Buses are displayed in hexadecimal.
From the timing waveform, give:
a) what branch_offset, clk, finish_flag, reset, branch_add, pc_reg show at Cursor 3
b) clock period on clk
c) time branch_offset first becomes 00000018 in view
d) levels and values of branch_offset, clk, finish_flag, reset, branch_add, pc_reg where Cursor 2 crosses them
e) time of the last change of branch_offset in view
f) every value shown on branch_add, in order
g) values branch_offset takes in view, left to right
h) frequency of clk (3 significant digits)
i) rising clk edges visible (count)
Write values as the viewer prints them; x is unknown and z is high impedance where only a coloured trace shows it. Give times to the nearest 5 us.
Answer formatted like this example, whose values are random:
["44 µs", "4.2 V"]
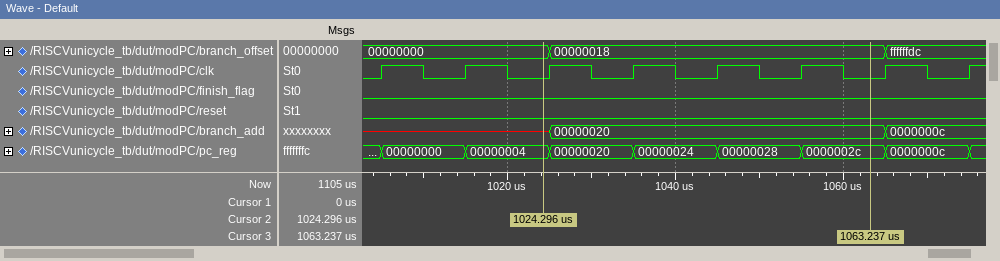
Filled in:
["branch_offset=00000018, clk=0, finish_flag=0, reset=0, branch_add=00000020, pc_reg=0000002c", "10 us", "1025 us", "branch_offset=00000000, clk=0, finish_flag=0, reset=0, branch_add=x, pc_reg=00000004", "1065 us", "x, 00000020, 0000000c", "00000000, 00000018, ffffffdc", "100 kHz", "8"]
